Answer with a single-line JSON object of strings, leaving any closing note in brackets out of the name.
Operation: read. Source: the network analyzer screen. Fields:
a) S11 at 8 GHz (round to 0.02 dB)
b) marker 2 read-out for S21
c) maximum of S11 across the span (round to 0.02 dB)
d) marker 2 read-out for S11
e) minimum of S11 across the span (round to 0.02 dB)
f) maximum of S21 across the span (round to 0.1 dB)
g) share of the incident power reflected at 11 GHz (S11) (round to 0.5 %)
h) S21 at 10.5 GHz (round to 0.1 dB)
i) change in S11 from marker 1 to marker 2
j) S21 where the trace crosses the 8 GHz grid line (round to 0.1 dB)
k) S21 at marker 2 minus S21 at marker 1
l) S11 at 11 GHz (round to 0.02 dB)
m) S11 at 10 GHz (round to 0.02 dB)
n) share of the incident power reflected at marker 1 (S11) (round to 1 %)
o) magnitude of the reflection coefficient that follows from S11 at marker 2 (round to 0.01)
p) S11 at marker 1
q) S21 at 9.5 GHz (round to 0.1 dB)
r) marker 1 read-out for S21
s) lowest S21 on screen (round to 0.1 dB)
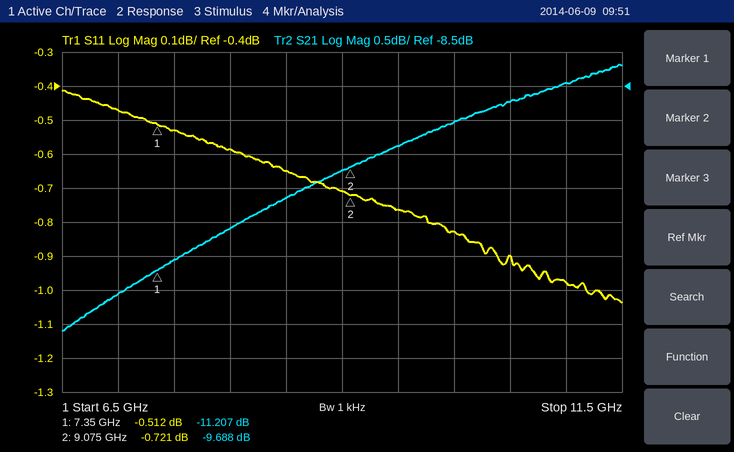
{"S11 at 8 GHz": "-0.58 dB", "marker 2 read-out for S21": "-9.688 dB", "maximum of S11 across the span": "-0.42 dB", "marker 2 read-out for S11": "-0.721 dB", "minimum of S11 across the span": "-1.04 dB", "maximum of S21 across the span": "-8.2 dB", "share of the incident power reflected at 11 GHz (S11)": "80.0 %", "S21 at 10.5 GHz": "-8.7 dB", "change in S11 from marker 1 to marker 2": "-0.209 dB", "S21 where the trace crosses the 8 GHz grid line": "-10.6 dB", "S21 at marker 2 minus S21 at marker 1": "1.519 dB", "S11 at 11 GHz": "-0.98 dB", "S11 at 10 GHz": "-0.82 dB", "share of the incident power reflected at marker 1 (S11)": "89 %", "magnitude of the reflection coefficient that follows from S11 at marker 2": "0.92", "S11 at marker 1": "-0.512 dB", "S21 at 9.5 GHz": "-9.4 dB", "marker 1 read-out for S21": "-11.207 dB", "lowest S21 on screen": "-12.1 dB"}
